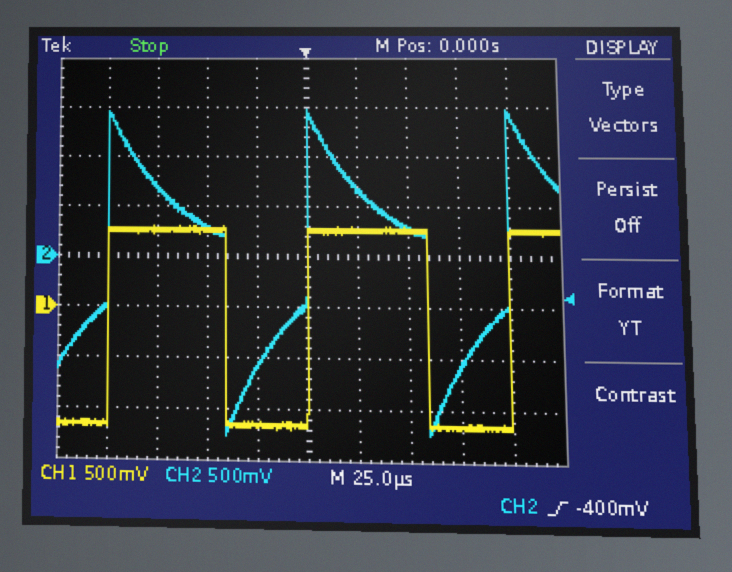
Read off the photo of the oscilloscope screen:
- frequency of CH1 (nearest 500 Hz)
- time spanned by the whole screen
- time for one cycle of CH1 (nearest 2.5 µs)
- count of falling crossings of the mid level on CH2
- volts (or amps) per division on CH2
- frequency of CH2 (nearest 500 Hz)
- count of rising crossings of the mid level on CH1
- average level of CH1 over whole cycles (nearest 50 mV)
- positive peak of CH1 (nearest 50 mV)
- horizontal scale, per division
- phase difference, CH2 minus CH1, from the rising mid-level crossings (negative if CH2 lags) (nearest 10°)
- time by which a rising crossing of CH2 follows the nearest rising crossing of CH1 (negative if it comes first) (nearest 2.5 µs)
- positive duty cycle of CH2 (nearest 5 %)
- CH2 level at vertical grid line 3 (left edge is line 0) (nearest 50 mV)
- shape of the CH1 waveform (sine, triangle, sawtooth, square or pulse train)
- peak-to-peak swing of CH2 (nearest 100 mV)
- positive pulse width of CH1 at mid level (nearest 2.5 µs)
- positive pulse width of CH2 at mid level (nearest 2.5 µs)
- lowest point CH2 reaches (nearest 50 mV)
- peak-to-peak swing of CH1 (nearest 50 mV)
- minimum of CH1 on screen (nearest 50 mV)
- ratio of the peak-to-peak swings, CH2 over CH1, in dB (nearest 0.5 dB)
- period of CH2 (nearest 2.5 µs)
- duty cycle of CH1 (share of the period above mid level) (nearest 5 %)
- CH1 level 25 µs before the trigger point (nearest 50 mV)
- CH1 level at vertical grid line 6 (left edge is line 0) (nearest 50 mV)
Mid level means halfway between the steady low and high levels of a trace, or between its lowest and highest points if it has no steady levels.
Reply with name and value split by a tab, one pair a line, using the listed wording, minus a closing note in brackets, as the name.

frequency of CH1	10.0 kHz
time spanned by the whole screen	250 µs
time for one cycle of CH1	100.0 µs
count of falling crossings of the mid level on CH2	2
volts (or amps) per division on CH2	500 mV
frequency of CH2	10.0 kHz
count of rising crossings of the mid level on CH1	3
average level of CH1 over whole cycles	0 mV
positive peak of CH1	800 mV
horizontal scale, per division	25 µs
phase difference, CH2 minus CH1, from the rising mid-level crossings (negative if CH2 lags)	0°
time by which a rising crossing of CH2 follows the nearest rising crossing of CH1 (negative if it comes first)	0.0 µs
positive duty cycle of CH2	60 %
CH2 level at vertical grid line 3 (left edge is line 0)	300 mV
shape of the CH1 waveform	pulse train
peak-to-peak swing of CH2	3.20 V
positive pulse width of CH1 at mid level	60.0 µs
positive pulse width of CH2 at mid level	60.0 µs
lowest point CH2 reaches	-1.75 V
peak-to-peak swing of CH1	2.00 V
minimum of CH1 on screen	-1.20 V
ratio of the peak-to-peak swings, CH2 over CH1, in dB	4.0 dB
period of CH2	100.0 µs
duty cycle of CH1 (share of the period above mid level)	60 %
CH1 level 25 µs before the trigger point	-1.15 V
CH1 level at vertical grid line 6 (left edge is line 0)	750 mV
